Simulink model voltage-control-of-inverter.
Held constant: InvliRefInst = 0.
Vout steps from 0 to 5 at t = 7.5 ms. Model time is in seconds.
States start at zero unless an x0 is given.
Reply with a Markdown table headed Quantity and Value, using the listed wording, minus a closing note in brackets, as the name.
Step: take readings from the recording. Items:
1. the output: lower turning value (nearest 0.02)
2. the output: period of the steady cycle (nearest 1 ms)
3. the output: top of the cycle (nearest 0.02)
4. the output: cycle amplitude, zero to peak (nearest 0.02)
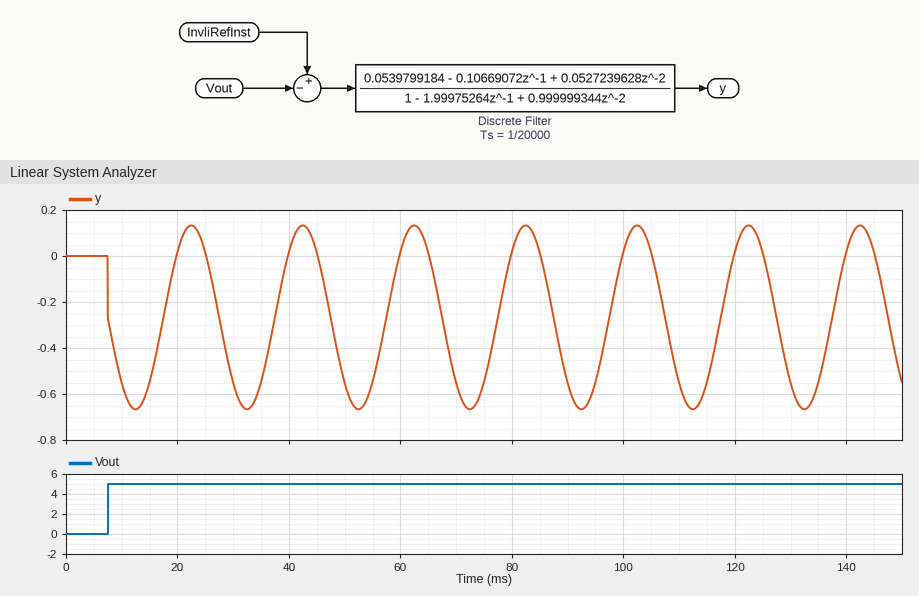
| Quantity | Value |
|---|---|
| the output: lower turning value | -0.66 |
| the output: period of the steady cycle | 20 ms |
| the output: top of the cycle | 0.14 |
| the output: cycle amplitude, zero to peak | 0.40 |
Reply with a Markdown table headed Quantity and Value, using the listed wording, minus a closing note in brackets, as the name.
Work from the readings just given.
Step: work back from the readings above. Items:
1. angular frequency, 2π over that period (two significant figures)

| Quantity | Value |
|---|---|
| angular frequency, 2π over that period | 0.31 rad/ms |
